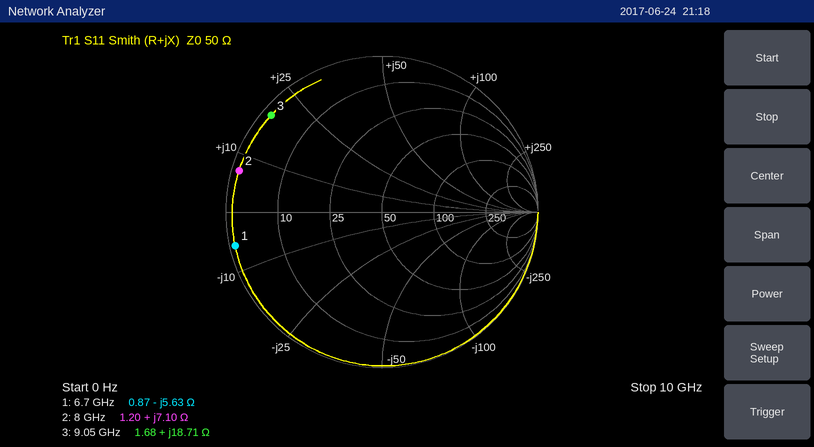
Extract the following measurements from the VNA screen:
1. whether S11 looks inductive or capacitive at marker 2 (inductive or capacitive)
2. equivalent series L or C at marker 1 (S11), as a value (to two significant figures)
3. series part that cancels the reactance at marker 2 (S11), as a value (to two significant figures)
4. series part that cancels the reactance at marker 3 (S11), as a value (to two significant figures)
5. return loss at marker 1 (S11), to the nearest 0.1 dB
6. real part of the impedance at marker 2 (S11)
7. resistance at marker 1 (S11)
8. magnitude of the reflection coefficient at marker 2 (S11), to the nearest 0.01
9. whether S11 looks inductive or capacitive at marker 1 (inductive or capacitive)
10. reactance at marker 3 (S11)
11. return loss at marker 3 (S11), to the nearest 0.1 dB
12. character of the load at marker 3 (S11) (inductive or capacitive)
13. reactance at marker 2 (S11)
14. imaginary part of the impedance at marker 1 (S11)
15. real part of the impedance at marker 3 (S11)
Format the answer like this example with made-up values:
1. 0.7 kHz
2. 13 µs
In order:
1. inductive
2. 4.2 pF
3. 2.8 pF
4. 940 fF
5. 0.3 dB
6. 1.20 Ω
7. 0.87 Ω
8. 0.95
9. capacitive
10. +18.71 Ω
11. 0.5 dB
12. inductive
13. +7.10 Ω
14. -5.63 Ω
15. 1.68 Ω
